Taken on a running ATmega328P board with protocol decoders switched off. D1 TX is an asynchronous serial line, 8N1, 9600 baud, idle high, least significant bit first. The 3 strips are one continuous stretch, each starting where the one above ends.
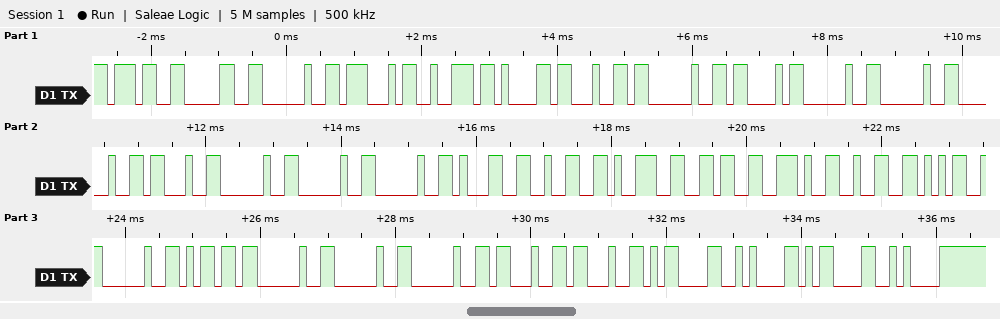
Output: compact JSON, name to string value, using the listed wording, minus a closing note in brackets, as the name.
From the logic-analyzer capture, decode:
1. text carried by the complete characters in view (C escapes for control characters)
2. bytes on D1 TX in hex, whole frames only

{"text carried by the complete characters in view": "\"70 Grad C   #   1296.25 m   ##\\r\\n\\r\\n\"", "bytes on D1 TX in hex, whole frames only": "37 30 20 47 72 61 64 20 43 20 20 20 23 20 20 20 31 32 39 36 2E 32 35 20 6D 20 20 20 23 23 0D 0A 0D 0A"}
